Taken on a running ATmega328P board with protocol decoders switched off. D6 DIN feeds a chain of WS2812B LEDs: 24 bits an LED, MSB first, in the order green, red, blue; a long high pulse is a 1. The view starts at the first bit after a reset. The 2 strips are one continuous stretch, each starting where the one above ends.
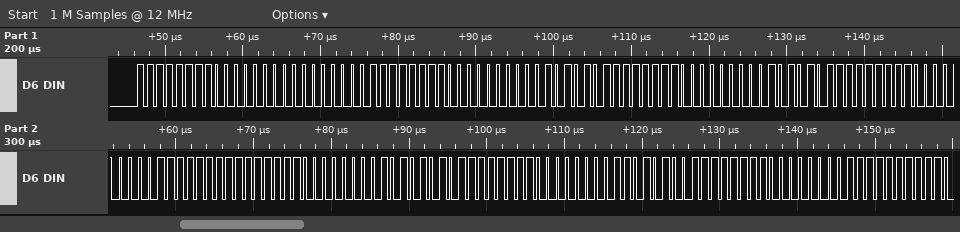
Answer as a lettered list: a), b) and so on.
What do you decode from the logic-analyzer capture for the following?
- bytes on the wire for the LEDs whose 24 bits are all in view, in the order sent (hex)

a) FF 00 00 FF 00 2A FF 00 55 FF 00 7F FF 00 AA FF 00 D4 FF 00 FF
